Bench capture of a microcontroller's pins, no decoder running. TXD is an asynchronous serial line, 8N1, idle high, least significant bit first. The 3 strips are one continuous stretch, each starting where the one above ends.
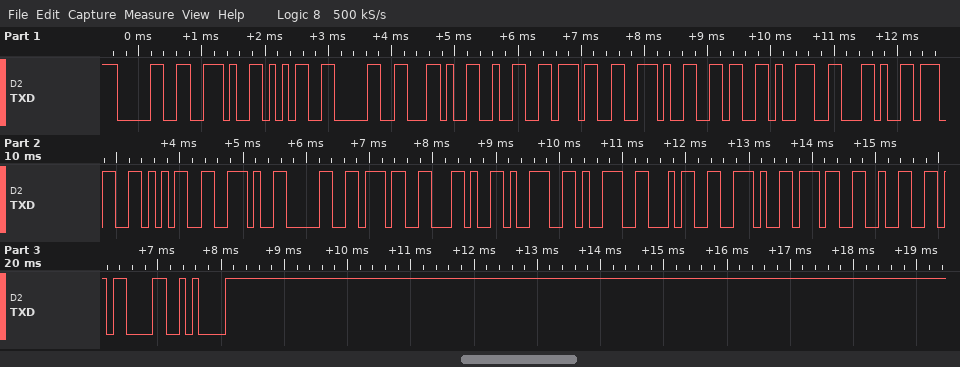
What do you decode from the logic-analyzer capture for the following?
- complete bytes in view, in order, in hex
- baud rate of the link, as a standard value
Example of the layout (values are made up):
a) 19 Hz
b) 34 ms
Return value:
a) 30 2E 35 30 2C 32 37 2E 36 39 2C 37 35 2E 30 37 2C 39 39 34 2E 37 32 0D 0A
b) 9600 baud
